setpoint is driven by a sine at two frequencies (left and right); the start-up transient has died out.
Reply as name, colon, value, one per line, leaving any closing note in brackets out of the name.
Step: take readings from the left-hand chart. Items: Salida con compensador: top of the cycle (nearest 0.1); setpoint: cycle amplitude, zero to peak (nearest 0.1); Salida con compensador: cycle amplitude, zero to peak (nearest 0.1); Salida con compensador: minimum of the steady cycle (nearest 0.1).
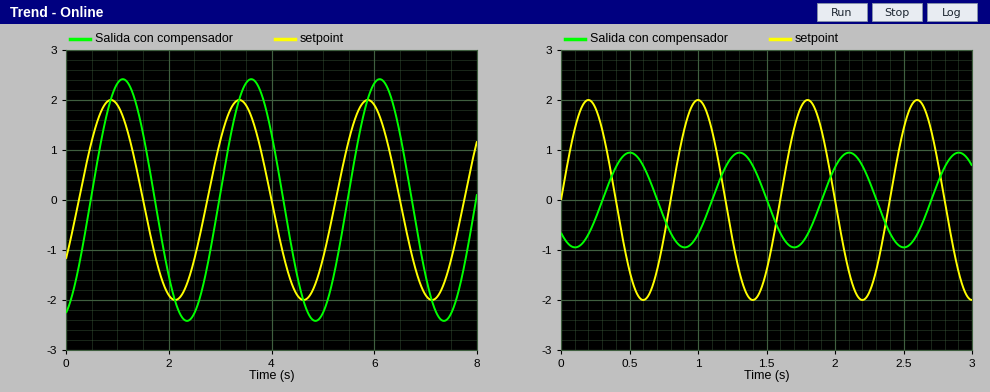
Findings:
Salida con compensador: top of the cycle: 2.4
setpoint: cycle amplitude, zero to peak: 2.0
Salida con compensador: cycle amplitude, zero to peak: 2.4
Salida con compensador: minimum of the steady cycle: -2.4
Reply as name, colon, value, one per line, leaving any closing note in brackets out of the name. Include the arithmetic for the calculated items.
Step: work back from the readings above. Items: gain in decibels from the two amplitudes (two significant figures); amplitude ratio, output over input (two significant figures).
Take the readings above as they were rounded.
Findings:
gain in decibels from the two amplitudes: 20 log10(2.4 / 2) = 1.6 dB
amplitude ratio, output over input: 2.4 / 2 = 1.2
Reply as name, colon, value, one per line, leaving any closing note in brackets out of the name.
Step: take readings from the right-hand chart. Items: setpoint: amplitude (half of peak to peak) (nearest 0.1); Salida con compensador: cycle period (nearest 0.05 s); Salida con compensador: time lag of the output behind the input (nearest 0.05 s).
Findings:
setpoint: amplitude (half of peak to peak): 2.0
Salida con compensador: cycle period: 0.80 s
Salida con compensador: time lag of the output behind the input: 0.30 s
